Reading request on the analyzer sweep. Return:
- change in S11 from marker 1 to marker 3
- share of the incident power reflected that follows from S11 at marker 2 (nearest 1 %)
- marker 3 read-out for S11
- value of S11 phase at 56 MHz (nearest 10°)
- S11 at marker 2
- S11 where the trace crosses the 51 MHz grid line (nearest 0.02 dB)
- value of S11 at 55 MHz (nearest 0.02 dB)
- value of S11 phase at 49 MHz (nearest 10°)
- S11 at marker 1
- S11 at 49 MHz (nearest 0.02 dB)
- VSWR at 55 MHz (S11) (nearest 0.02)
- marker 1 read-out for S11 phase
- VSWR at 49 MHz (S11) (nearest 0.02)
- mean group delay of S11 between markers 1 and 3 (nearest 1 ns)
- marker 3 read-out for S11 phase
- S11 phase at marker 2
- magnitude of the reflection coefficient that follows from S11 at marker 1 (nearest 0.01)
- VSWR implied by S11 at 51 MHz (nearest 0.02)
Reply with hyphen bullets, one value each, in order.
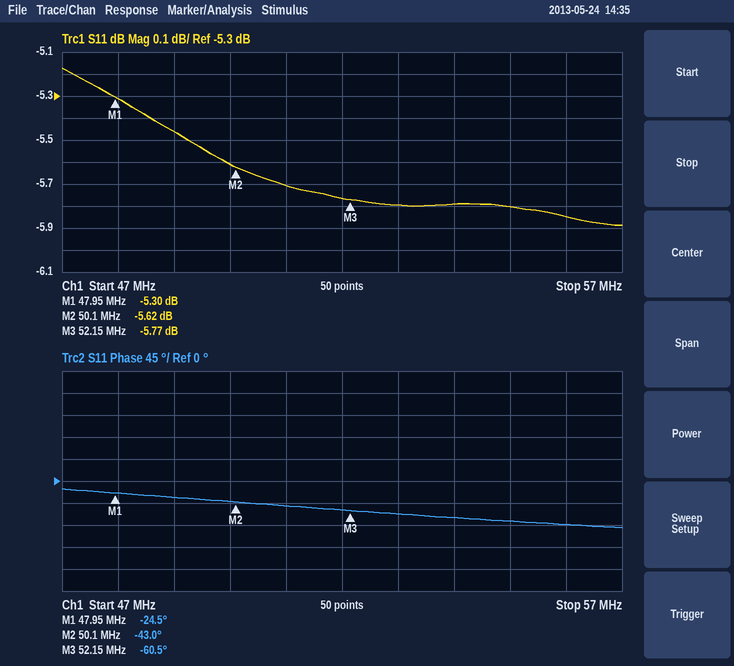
- -0.47 dB
- 27 %
- -5.77 dB
- -90°
- -5.62 dB
- -5.70 dB
- -5.80 dB
- -30°
- -5.30 dB
- -5.46 dB
- 3.10
- -24.5°
- 3.28
- 24 ns
- -60.5°
- -43.0°
- 0.54
- 3.16
